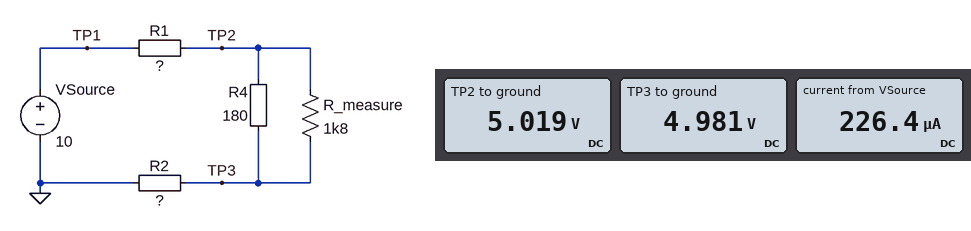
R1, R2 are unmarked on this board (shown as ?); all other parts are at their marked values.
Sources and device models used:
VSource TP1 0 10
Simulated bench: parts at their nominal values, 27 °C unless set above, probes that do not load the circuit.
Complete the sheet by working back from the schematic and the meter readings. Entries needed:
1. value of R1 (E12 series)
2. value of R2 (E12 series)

22 kΩ
22 kΩ
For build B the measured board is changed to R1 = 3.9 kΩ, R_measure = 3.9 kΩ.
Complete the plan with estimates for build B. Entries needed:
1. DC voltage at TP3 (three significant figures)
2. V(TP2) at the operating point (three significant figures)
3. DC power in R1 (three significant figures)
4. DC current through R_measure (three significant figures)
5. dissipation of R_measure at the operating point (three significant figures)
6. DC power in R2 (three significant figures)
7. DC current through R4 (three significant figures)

8.44 V
8.50 V
574 µW
16.9 µA
1.12 µW
3.24 mW
367 µA
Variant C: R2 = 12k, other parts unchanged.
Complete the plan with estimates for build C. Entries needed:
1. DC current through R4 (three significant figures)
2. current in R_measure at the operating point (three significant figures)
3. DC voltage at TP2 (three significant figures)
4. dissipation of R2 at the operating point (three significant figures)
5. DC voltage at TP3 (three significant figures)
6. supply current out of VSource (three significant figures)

266 µA
26.6 µA
3.56 V
1.03 mW
3.51 V
293 µA
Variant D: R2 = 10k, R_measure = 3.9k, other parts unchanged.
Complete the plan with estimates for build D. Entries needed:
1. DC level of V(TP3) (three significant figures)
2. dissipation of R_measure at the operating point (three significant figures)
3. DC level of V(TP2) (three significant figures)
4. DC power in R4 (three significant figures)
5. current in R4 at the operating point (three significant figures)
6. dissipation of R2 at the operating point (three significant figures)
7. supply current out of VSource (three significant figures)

3.11 V
733 nW
3.16 V
15.9 µW
297 µA
966 µW
311 µA
